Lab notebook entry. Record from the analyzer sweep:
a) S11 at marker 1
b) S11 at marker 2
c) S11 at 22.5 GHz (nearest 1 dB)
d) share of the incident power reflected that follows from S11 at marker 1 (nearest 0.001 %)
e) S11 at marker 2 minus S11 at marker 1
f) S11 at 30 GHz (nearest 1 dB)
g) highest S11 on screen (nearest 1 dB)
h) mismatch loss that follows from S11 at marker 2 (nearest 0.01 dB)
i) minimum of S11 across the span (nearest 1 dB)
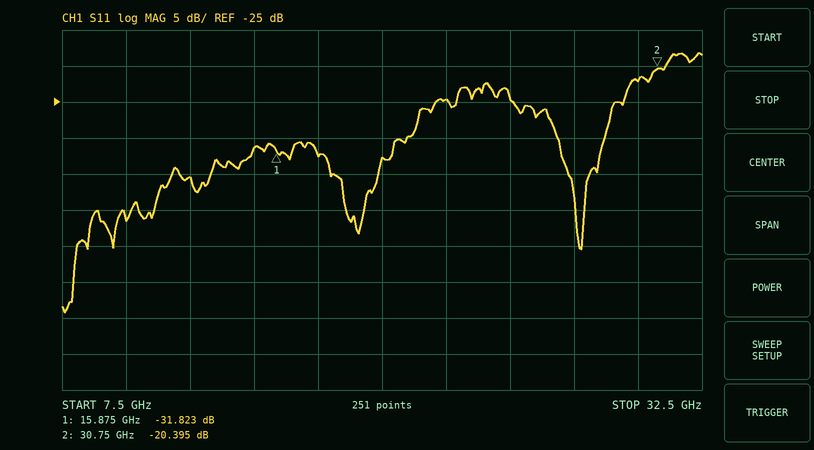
-31.823 dB
-20.395 dB
-25 dB
0.066 %
11.428 dB
-22 dB
-18 dB
0.04 dB
-54 dB
